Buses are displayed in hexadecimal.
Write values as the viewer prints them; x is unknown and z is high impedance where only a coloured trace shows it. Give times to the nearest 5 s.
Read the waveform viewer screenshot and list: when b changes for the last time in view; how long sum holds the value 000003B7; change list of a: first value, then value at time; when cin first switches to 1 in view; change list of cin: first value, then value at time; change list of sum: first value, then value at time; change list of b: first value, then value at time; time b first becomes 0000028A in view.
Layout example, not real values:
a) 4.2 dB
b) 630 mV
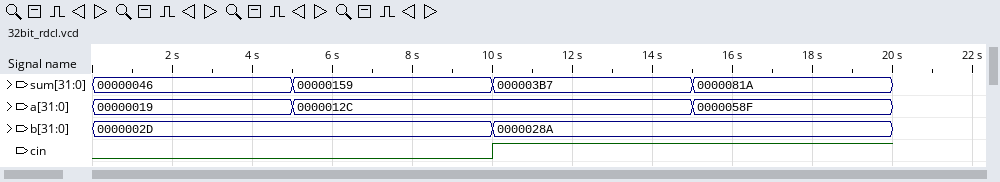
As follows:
a) 10 s
b) 5 s
c) 00000019, 0000012C at 5 s, 0000058F at 15 s
d) 10 s
e) 0, 1 at 10 s
f) 00000046, 00000159 at 5 s, 000003B7 at 10 s, 0000081A at 15 s
g) 0000002D, 0000028A at 10 s
h) 10 s
